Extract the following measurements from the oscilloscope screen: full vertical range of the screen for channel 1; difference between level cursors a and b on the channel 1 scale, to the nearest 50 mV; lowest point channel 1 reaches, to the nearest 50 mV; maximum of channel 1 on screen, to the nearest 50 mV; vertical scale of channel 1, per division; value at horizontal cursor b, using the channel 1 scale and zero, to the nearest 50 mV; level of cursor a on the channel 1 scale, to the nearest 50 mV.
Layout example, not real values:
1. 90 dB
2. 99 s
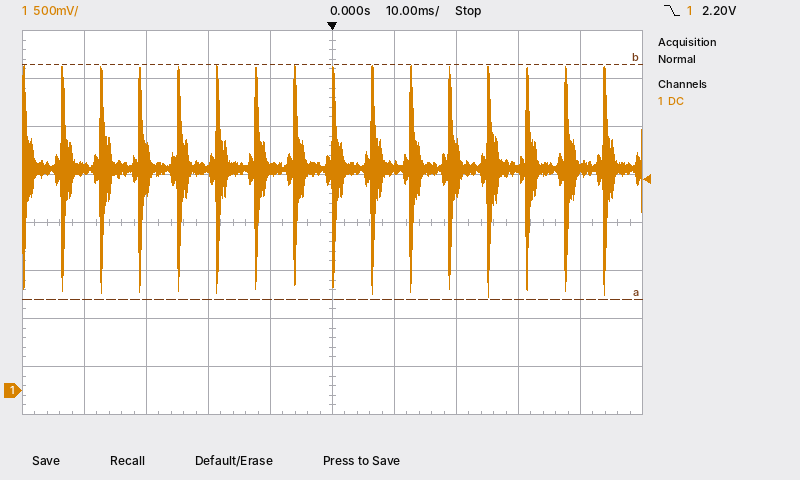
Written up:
1. 4 V
2. 2.45 V
3. 950 mV
4. 3.40 V
5. 500 mV
6. 3.40 V
7. 950 mV
